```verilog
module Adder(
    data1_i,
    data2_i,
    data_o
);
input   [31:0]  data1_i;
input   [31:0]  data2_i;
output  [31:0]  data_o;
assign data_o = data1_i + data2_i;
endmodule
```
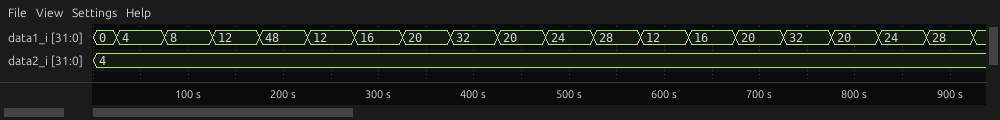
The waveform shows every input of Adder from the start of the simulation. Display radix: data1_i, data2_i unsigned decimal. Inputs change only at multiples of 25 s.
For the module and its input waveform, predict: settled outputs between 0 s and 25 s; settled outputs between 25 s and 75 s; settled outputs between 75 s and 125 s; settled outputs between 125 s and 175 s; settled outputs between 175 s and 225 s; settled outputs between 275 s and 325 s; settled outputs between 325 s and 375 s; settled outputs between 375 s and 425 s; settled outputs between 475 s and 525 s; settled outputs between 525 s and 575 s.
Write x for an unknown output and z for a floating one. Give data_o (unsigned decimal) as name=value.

data_o=4
data_o=8
data_o=12
data_o=16
data_o=52
data_o=20
data_o=24
data_o=36
data_o=28
data_o=32
